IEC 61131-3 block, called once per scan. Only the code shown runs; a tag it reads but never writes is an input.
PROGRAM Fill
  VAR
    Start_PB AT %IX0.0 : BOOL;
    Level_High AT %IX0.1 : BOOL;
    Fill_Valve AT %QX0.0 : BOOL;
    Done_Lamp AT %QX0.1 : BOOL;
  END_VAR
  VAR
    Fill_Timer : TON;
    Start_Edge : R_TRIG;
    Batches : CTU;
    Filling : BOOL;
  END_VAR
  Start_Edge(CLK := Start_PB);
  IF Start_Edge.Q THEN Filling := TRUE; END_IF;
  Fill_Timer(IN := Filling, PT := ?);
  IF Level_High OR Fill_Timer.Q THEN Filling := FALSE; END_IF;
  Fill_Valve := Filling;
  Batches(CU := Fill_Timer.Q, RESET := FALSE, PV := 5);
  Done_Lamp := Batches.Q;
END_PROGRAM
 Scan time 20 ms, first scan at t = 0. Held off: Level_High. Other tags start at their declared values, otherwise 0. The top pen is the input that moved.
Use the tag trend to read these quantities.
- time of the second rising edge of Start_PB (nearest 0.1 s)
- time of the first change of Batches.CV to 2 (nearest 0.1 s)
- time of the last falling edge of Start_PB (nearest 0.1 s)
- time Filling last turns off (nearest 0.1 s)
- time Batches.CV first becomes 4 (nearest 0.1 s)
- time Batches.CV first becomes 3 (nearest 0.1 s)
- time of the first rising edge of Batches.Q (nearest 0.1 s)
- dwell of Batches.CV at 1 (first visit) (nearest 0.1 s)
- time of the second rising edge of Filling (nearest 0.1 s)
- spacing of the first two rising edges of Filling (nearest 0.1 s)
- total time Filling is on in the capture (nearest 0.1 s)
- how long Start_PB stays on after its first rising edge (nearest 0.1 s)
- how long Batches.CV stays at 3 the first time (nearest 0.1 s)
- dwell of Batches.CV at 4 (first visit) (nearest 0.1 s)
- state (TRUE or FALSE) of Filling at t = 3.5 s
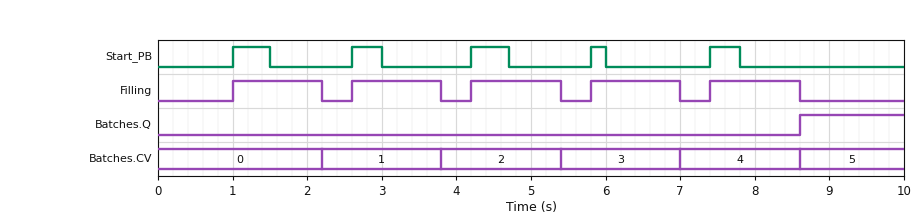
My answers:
2.6 s
3.8 s
7.8 s
8.6 s
7.0 s
5.4 s
8.6 s
1.6 s
2.6 s
1.6 s
6.0 s
0.5 s
1.6 s
1.6 s
TRUE
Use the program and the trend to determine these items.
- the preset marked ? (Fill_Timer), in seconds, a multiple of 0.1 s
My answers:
1.2 s
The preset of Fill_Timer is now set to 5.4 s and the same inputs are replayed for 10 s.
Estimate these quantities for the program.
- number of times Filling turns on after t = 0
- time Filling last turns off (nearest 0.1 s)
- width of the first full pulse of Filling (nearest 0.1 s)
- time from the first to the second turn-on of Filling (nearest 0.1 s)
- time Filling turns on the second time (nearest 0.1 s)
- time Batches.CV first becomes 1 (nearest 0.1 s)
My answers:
2
6.4 s
5.4 s
6.4 s
7.4 s
6.4 s
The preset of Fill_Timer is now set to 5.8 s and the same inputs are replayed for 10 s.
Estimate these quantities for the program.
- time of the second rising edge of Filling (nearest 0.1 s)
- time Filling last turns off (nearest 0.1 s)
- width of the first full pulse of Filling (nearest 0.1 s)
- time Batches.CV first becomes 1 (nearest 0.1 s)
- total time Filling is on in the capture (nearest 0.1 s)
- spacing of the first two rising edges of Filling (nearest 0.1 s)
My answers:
7.4 s
6.8 s
5.8 s
6.8 s
8.4 s
6.4 s
